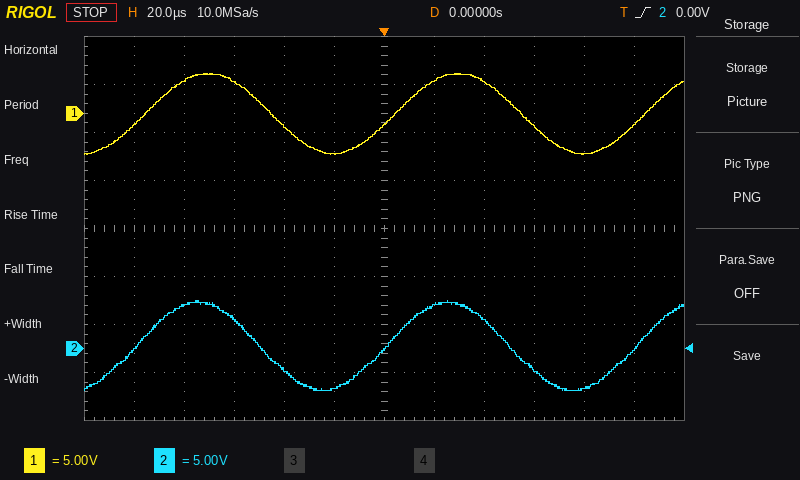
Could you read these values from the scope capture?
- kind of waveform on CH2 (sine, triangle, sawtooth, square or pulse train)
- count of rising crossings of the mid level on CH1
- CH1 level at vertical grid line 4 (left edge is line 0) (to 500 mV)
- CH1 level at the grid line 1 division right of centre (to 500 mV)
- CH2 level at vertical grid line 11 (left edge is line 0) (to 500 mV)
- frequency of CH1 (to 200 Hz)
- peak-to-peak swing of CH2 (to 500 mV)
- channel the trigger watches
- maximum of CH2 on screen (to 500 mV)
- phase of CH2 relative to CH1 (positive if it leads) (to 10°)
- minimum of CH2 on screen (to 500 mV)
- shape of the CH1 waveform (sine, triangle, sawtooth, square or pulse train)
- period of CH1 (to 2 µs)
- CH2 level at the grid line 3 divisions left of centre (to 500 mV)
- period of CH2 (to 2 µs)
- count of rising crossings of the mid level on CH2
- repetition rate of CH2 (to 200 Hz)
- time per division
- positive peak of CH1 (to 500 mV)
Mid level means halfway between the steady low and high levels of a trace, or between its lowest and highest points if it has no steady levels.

sine
3
-1.5 V
3.5 V
0.0 V
10.0 kHz
9.5 V
CH2
5.0 V
+10°
-4.5 V
sine
100 µs
3.0 V
100 µs
3
10.0 kHz
20 µs
4.0 V
